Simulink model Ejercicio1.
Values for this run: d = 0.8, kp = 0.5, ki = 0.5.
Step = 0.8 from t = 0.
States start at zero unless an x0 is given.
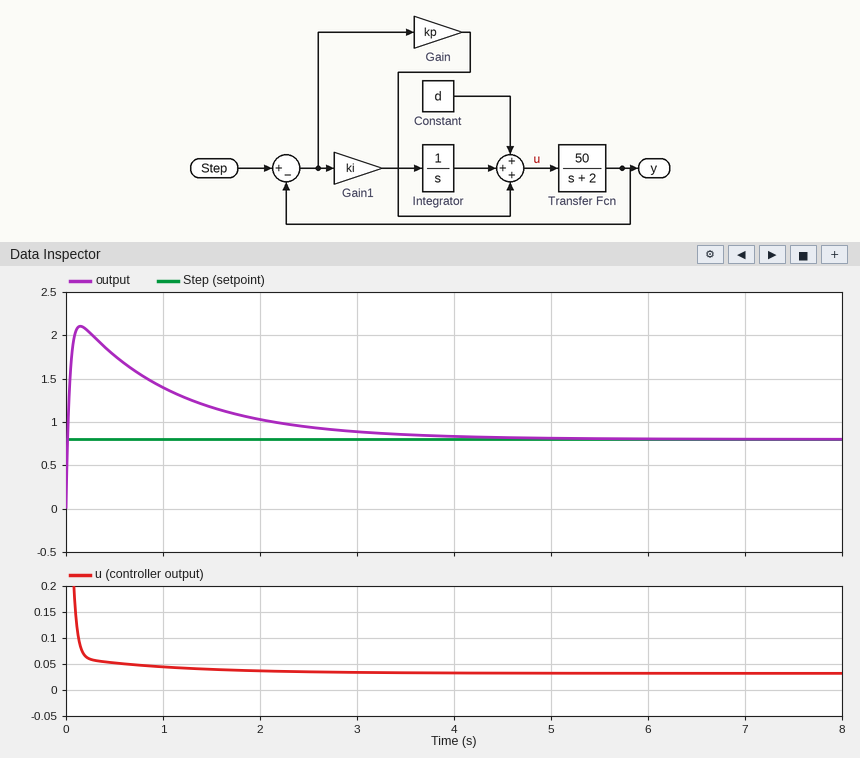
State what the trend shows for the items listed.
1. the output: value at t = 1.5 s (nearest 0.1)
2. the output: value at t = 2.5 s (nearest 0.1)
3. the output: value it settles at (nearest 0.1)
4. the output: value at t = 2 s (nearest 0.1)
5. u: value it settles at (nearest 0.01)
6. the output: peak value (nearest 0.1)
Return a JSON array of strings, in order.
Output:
["1.2", "0.9", "0.8", "1.0", "0.03", "2.1"]
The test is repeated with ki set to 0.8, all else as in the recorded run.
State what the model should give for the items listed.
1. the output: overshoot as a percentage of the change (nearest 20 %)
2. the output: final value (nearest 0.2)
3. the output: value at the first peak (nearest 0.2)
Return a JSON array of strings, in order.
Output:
["160 %", "0.8", "2.0"]
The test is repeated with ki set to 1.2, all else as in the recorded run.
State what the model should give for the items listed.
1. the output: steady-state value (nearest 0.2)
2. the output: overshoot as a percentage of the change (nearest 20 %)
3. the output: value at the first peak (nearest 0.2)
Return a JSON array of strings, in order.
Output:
["0.8", "160 %", "2.0"]
